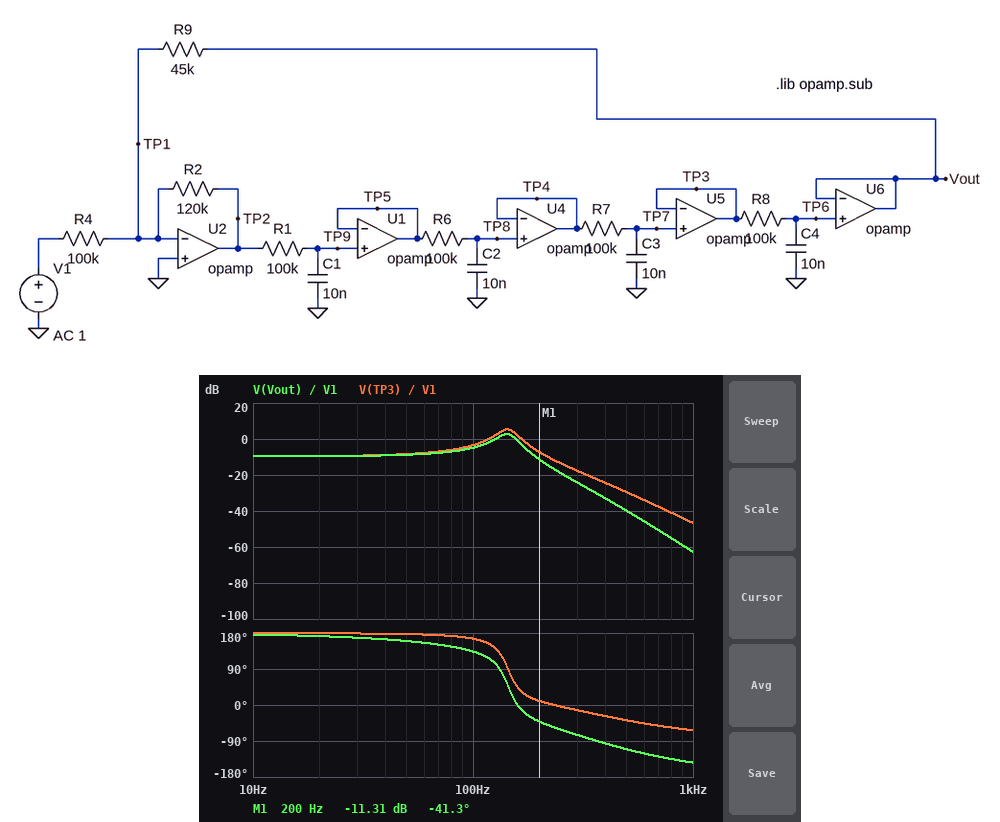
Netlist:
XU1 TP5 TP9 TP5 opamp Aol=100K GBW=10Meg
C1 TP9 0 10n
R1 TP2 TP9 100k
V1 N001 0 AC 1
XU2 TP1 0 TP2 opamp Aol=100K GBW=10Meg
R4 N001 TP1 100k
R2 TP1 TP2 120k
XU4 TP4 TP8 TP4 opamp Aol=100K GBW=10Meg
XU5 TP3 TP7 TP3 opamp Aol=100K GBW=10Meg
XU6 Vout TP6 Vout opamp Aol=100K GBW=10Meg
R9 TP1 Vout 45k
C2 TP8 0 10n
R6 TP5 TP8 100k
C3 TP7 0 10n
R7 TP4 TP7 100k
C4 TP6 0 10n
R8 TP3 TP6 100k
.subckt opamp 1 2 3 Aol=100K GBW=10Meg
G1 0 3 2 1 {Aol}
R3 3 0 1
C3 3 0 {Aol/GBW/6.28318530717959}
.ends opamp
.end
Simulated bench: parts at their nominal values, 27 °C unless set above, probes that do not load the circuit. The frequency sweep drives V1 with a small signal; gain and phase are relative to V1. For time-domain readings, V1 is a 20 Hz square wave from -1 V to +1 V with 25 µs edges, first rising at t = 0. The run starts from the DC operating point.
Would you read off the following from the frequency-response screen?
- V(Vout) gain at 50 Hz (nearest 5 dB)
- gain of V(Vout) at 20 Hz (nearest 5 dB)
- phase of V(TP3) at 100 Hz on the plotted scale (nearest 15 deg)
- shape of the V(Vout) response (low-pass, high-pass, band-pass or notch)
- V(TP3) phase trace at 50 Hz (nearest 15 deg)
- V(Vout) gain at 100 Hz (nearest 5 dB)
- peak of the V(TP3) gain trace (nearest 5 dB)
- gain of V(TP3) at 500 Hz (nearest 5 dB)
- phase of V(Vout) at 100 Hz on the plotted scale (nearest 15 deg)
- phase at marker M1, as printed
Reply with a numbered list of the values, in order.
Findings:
1. -10 dB
2. -10 dB
3. 165 deg
4. low-pass
5. 180 deg
6. -5 dB
7. 5 dB
8. -30 dB
9. 135 deg
10. -41.3 deg
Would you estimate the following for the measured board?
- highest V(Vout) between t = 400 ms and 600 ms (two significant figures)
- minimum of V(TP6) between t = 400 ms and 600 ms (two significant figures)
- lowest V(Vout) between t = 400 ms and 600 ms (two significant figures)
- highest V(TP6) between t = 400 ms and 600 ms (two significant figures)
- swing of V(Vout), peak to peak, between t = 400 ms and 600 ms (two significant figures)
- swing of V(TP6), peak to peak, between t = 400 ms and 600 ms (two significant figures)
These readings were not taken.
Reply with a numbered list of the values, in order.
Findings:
1. 780 mV
2. -780 mV
3. -780 mV
4. 780 mV
5. 1.6 V
6. 1.6 V
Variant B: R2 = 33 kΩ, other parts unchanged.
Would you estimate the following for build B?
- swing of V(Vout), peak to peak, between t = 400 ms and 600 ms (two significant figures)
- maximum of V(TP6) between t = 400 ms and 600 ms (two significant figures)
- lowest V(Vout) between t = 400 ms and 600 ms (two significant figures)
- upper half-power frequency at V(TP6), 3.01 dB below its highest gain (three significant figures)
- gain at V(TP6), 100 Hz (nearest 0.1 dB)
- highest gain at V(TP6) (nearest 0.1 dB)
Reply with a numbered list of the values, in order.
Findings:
1. 510 mV
2. 250 mV
3. -250 mV
4. 131 Hz
5. -13.7 dB
6. -13.3 dB
